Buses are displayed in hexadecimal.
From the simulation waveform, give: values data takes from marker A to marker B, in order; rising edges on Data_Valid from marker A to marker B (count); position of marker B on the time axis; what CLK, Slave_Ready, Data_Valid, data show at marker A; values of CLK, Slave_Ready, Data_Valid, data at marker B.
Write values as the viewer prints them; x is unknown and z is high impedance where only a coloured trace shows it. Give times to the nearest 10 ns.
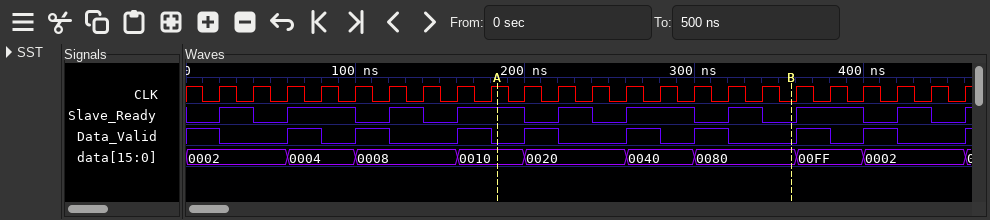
0010, 0020, 0040, 0080
3
360 ns
CLK=1, Slave_Ready=1, Data_Valid=0, data=0010
CLK=0, Slave_Ready=0, Data_Valid=0, data=0080
